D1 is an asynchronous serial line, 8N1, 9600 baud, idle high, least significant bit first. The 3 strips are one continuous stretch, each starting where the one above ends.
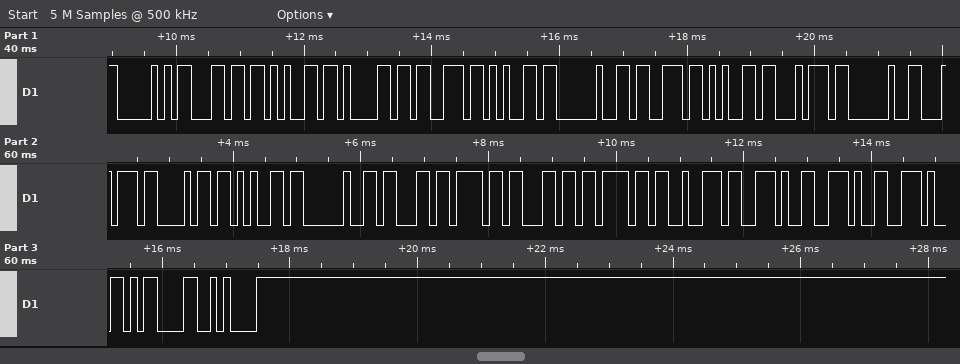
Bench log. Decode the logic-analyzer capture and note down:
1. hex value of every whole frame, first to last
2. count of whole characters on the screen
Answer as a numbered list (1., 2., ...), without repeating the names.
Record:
1. 50 6C 65 61 73 65 20 73 65 74 20 74 68 65 20 63 6F 6C 6F 72 2E 2E 2E 0D 0A
2. 25
